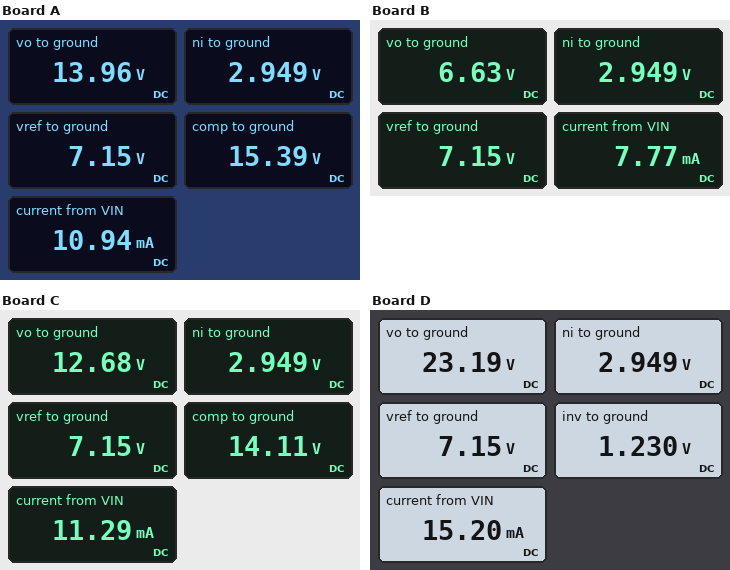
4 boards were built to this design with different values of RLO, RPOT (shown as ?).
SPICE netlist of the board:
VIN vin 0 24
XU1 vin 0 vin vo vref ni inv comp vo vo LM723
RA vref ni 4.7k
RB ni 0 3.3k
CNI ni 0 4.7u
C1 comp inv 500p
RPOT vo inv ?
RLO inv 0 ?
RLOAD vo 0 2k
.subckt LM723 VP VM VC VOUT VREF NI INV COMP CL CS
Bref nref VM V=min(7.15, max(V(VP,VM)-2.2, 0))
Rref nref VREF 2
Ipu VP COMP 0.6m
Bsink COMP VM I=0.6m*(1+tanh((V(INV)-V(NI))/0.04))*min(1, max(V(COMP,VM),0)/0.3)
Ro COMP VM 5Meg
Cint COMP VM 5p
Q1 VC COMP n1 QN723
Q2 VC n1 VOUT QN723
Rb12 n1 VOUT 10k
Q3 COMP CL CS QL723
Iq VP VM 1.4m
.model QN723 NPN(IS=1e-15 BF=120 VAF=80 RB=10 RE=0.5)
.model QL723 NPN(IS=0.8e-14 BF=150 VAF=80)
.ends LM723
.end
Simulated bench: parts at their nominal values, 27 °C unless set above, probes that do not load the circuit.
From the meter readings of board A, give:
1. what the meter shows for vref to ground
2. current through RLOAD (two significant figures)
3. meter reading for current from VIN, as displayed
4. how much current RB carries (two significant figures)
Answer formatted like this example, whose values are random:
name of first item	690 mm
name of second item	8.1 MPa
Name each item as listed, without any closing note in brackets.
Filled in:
what the meter shows for vref to ground	7.15 V
current through RLOAD	7.0 mA
meter reading for current from VIN, as displayed	10.94 mA
how much current RB carries	890 µA
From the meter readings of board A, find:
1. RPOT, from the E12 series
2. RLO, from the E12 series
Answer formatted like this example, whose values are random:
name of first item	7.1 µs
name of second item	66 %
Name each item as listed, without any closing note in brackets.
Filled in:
RPOT, from the E12 series	5.6 kΩ
RLO, from the E12 series	1.5 kΩ
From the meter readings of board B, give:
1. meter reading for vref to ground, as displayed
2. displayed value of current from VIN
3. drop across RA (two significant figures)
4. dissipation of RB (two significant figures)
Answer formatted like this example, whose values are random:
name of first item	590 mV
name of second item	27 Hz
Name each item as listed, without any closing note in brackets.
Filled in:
meter reading for vref to ground, as displayed	7.15 V
displayed value of current from VIN	7.77 mA
drop across RA	4.2 V
dissipation of RB	2.6 mW
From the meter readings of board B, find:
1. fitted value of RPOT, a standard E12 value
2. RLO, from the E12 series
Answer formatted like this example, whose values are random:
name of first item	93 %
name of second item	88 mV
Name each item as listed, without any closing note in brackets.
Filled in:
fitted value of RPOT, a standard E12 value	1.5 kΩ
RLO, from the E12 series	1.2 kΩ
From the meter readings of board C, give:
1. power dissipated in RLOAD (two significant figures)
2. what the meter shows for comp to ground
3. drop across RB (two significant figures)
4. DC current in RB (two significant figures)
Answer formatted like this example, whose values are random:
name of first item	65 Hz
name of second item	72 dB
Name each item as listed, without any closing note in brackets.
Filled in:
power dissipated in RLOAD	80 mW
what the meter shows for comp to ground	14.11 V
drop across RB	2.9 V
DC current in RB	890 µA
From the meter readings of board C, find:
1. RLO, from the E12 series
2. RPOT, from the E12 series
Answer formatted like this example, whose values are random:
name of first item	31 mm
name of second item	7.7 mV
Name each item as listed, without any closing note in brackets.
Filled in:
RLO, from the E12 series	1 kΩ
RPOT, from the E12 series	3.3 kΩ
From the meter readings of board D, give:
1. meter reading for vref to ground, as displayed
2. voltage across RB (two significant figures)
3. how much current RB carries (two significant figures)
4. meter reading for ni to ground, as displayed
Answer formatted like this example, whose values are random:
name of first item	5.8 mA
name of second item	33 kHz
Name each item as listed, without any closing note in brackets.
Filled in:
meter reading for vref to ground, as displayed	7.15 V
voltage across RB	2.9 V
how much current RB carries	890 µA
meter reading for ni to ground, as displayed	2.949 V
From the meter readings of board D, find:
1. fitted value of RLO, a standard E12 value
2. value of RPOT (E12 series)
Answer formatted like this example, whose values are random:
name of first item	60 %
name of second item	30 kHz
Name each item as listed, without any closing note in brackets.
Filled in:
fitted value of RLO, a standard E12 value	560 Ω
value of RPOT	10 kΩ
